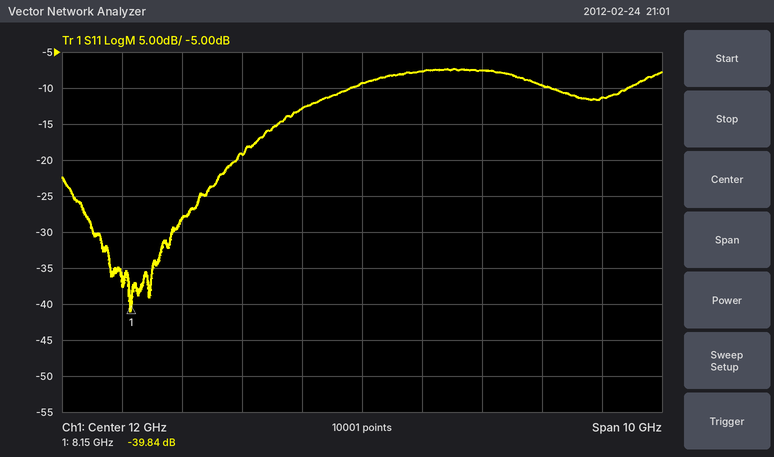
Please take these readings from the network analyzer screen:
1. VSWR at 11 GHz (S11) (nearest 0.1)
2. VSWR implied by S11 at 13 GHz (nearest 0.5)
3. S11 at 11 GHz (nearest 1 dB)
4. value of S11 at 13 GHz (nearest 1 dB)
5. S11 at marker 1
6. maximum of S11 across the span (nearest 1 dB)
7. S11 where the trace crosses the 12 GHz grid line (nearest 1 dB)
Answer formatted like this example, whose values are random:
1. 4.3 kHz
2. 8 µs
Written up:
1. 1.6
2. 2.5
3. -13 dB
4. -8 dB
5. -39.84 dB
6. -7 dB
7. -9 dB
